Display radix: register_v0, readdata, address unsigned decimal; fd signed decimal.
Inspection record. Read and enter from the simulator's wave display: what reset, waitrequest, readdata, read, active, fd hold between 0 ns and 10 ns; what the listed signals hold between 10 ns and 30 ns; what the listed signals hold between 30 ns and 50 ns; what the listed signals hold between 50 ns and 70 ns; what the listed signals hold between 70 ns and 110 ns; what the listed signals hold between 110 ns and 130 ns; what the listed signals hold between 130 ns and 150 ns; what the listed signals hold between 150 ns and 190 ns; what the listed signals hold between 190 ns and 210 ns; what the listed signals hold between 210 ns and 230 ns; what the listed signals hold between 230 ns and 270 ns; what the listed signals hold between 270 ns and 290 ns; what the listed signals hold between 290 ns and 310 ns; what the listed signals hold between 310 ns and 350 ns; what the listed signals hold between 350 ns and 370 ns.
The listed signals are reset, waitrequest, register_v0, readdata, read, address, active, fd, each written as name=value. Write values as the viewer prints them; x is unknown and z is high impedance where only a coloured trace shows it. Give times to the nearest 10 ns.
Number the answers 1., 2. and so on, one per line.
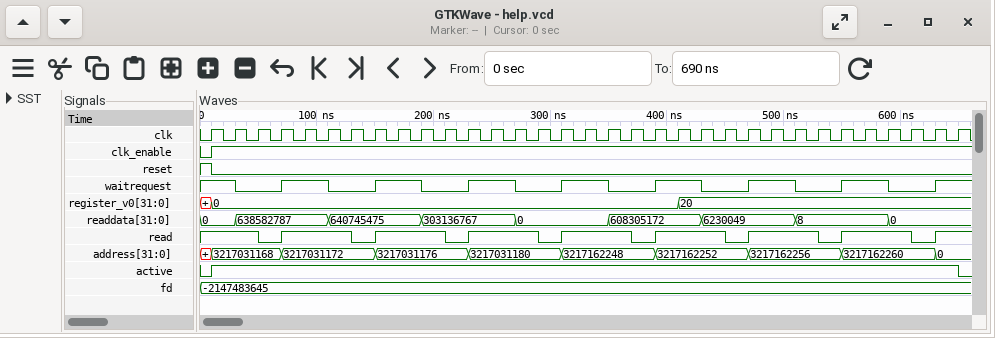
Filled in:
1. reset=1, waitrequest=1, readdata=0, read=1, active=0, fd=-2147483645
2. reset=0, waitrequest=1, register_v0=0, readdata=0, read=1, address=3217031168, active=1, fd=-2147483645
3. reset=0, waitrequest=0, register_v0=0, readdata=638582787, read=1, address=3217031168, active=1, fd=-2147483645
4. reset=0, waitrequest=0, register_v0=0, readdata=638582787, read=0, address=3217031168, active=1, fd=-2147483645
5. reset=0, waitrequest=1, register_v0=0, readdata=638582787, read=1, address=3217031172, active=1, fd=-2147483645
6. reset=0, waitrequest=0, register_v0=0, readdata=640745475, read=1, address=3217031172, active=1, fd=-2147483645
7. reset=0, waitrequest=0, register_v0=0, readdata=640745475, read=0, address=3217031172, active=1, fd=-2147483645
8. reset=0, waitrequest=1, register_v0=0, readdata=640745475, read=1, address=3217031176, active=1, fd=-2147483645
9. reset=0, waitrequest=0, register_v0=0, readdata=303136767, read=1, address=3217031176, active=1, fd=-2147483645
10. reset=0, waitrequest=0, register_v0=0, readdata=303136767, read=0, address=3217031176, active=1, fd=-2147483645
11. reset=0, waitrequest=1, register_v0=0, readdata=303136767, read=1, address=3217031180, active=1, fd=-2147483645
12. reset=0, waitrequest=0, register_v0=0, readdata=0, read=1, address=3217031180, active=1, fd=-2147483645
13. reset=0, waitrequest=0, register_v0=0, readdata=0, read=0, address=3217031180, active=1, fd=-2147483645
14. reset=0, waitrequest=1, register_v0=0, readdata=0, read=1, address=3217162248, active=1, fd=-2147483645
15. reset=0, waitrequest=0, register_v0=0, readdata=608305172, read=1, address=3217162248, active=1, fd=-2147483645
